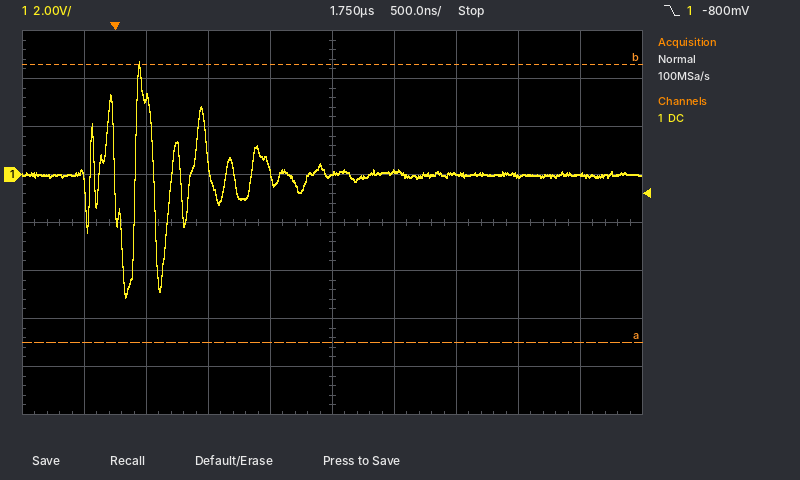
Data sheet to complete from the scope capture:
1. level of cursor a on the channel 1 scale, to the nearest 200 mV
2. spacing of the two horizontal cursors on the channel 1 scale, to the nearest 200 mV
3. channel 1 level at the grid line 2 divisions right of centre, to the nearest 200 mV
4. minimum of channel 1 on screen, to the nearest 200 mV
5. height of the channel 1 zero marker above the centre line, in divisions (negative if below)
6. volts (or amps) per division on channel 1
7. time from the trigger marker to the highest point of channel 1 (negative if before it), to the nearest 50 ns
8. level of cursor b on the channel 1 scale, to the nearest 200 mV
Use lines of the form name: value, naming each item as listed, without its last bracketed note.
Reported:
level of cursor a on the channel 1 scale, to the nearest 200 mV: -7.0 V
spacing of the two horizontal cursors on the channel 1 scale, to the nearest 200 mV: 11.6 V
channel 1 level at the grid line 2 divisions right of centre, to the nearest 200 mV: 0.0 V
minimum of channel 1 on screen, to the nearest 200 mV: -5.2 V
height of the channel 1 zero marker above the centre line, in divisions: +1.0 div
volts (or amps) per division on channel 1: 2 V
time from the trigger marker to the highest point of channel 1 (negative if before it), to the nearest 50 ns: +200 ns
level of cursor b on the channel 1 scale, to the nearest 200 mV: 4.6 V
